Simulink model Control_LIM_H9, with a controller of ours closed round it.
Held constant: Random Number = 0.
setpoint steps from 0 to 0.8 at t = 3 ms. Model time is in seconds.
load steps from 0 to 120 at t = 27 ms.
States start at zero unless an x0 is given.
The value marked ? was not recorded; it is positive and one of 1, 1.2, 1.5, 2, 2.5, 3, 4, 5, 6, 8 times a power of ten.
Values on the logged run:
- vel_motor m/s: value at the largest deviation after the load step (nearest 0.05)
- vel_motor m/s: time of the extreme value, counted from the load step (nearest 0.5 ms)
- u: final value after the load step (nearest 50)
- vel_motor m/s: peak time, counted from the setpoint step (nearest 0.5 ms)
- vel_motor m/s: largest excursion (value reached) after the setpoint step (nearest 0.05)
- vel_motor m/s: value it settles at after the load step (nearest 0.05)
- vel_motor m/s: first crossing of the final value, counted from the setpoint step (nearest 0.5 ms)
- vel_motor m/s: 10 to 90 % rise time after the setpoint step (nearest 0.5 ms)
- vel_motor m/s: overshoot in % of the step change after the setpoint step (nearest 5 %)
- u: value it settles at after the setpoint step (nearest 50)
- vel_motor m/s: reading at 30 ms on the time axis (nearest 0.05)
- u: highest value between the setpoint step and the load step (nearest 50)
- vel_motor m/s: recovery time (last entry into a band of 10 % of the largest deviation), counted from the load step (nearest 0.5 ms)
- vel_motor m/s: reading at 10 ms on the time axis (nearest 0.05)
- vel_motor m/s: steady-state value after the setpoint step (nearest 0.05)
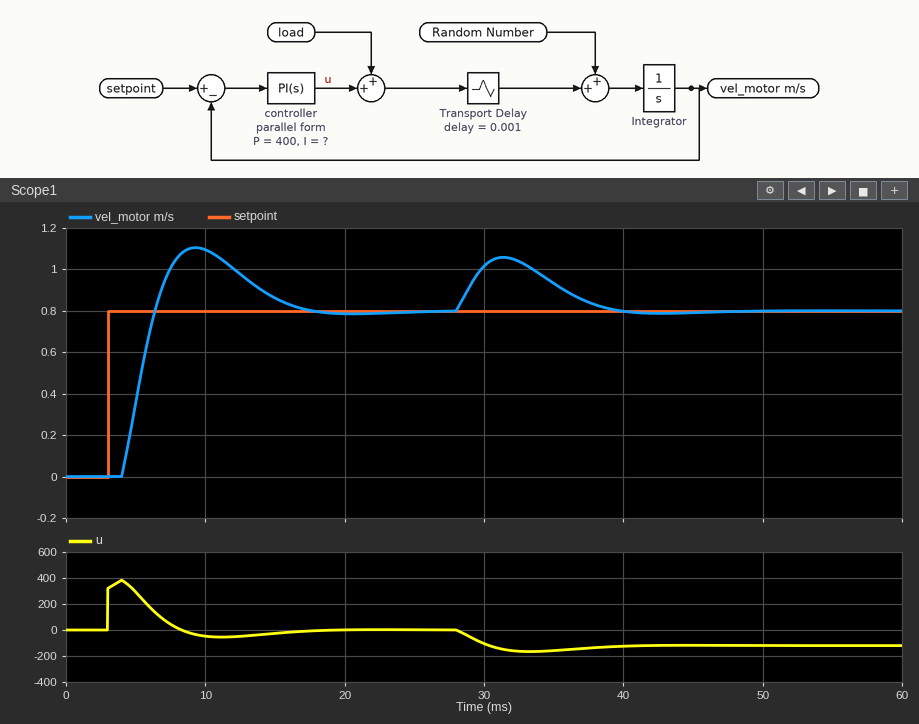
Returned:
1.05
4.5 ms
-100
6.5 ms
1.10
0.80
3.5 ms
2.0 ms
40 %
0
1.00
400
11.0 ms
1.10
0.80
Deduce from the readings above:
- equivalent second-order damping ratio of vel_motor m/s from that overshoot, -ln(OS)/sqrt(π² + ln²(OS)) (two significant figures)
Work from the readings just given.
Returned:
0.28
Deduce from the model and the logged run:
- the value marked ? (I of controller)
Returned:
80000
